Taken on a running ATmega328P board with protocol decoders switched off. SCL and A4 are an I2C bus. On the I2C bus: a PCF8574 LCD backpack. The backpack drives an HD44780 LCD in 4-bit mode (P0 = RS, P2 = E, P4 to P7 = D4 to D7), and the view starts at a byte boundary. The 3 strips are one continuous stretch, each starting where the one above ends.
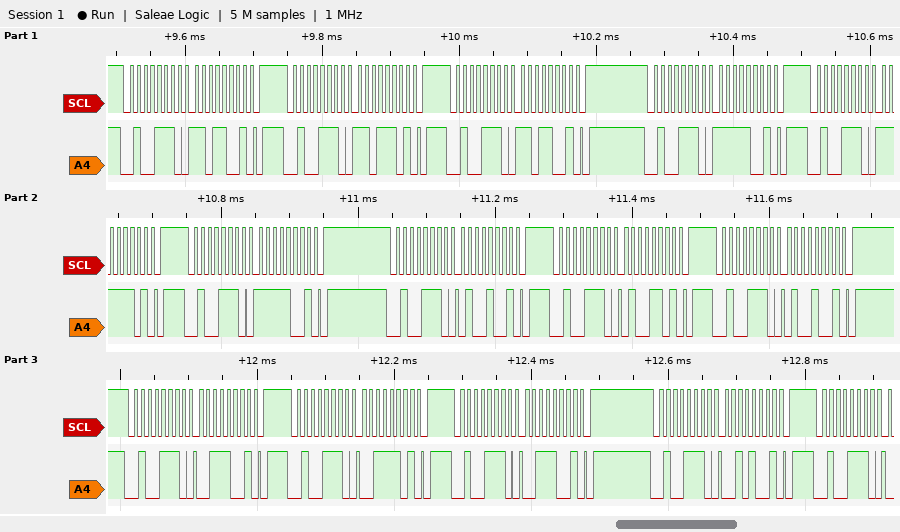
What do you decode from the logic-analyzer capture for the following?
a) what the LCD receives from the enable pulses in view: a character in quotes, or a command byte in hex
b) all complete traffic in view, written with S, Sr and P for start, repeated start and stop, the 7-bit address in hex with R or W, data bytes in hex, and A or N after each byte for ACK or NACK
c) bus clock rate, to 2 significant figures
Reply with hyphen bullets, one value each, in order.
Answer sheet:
- data 0xDF 'C'
- S 27W A D9 A P S 27W A DD A P S 27W A D9 A P S 27W A F9 A P S 27W A FD A P S 27W A F9 A P S 27W A 49 A P S 27W A 4D A P S 27W A 49 A P S 27W A 39 A P S 27W A 3D A P S 27W A 39 A P S 27W A 29 A P S 27W A
- 100 kHz
